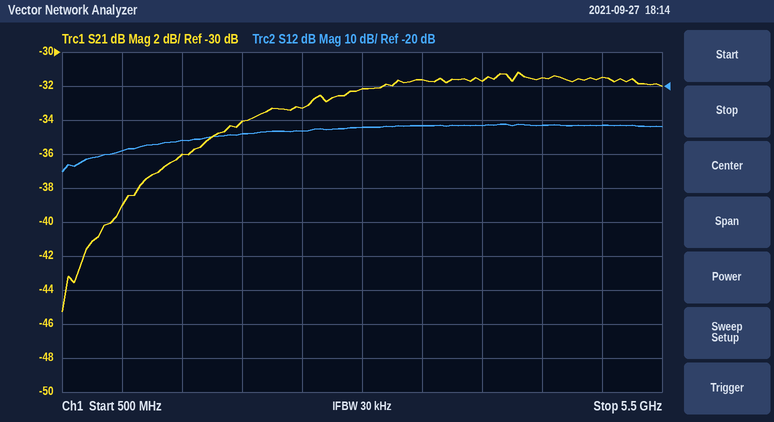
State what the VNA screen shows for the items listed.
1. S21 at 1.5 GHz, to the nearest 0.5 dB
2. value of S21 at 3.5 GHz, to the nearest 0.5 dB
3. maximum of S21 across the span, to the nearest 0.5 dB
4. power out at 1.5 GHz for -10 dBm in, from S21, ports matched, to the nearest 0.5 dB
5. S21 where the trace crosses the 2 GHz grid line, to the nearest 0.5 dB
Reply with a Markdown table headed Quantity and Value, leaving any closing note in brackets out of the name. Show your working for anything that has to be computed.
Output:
| Quantity | Value |
|---|---|
| S21 at 1.5 GHz, to the nearest 0.5 dB | -36.0 dB |
| value of S21 at 3.5 GHz, to the nearest 0.5 dB | -31.5 dB |
| maximum of S21 across the span, to the nearest 0.5 dB | -31.0 dB |
| power out at 1.5 GHz for -10 dBm in, from S21, ports matched, to the nearest 0.5 dB | -10 dBm + (-36.0 dB) = -46.0 dBm |
| S21 where the trace crosses the 2 GHz grid line, to the nearest 0.5 dB | -34.0 dB |
